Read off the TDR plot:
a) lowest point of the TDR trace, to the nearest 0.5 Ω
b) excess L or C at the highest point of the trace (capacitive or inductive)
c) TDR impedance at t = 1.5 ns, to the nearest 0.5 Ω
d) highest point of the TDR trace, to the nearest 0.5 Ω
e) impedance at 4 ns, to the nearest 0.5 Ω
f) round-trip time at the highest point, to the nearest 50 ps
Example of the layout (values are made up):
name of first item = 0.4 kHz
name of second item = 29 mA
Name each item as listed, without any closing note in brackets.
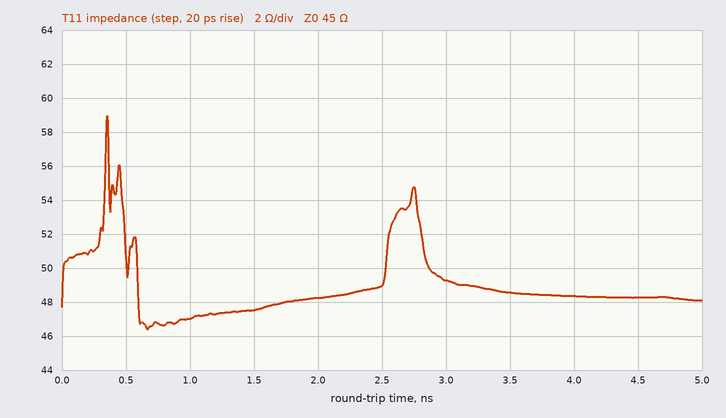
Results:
lowest point of the TDR trace, to the nearest 0.5 Ω = 46.5 Ω
excess L or C at the highest point of the trace = inductive
TDR impedance at t = 1.5 ns, to the nearest 0.5 Ω = 47.5 Ω
highest point of the TDR trace, to the nearest 0.5 Ω = 59.0 Ω
impedance at 4 ns, to the nearest 0.5 Ω = 48.5 Ω
round-trip time at the highest point, to the nearest 50 ps = 350 ps
